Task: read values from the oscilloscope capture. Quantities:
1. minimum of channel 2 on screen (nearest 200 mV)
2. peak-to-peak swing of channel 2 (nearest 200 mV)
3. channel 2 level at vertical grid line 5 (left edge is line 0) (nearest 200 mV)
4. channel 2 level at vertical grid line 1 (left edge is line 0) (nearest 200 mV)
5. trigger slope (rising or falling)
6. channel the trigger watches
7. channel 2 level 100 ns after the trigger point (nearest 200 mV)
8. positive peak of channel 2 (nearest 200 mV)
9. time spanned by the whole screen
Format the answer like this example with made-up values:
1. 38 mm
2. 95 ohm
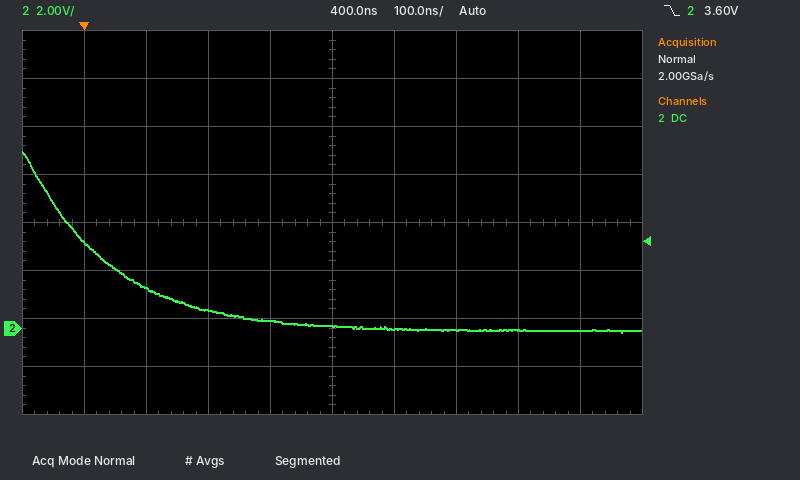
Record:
1. -200 mV
2. 7.6 V
3. 0.0 V
4. 3.6 V
5. falling
6. channel 2
7. 1.6 V
8. 7.4 V
9. 1 µs
